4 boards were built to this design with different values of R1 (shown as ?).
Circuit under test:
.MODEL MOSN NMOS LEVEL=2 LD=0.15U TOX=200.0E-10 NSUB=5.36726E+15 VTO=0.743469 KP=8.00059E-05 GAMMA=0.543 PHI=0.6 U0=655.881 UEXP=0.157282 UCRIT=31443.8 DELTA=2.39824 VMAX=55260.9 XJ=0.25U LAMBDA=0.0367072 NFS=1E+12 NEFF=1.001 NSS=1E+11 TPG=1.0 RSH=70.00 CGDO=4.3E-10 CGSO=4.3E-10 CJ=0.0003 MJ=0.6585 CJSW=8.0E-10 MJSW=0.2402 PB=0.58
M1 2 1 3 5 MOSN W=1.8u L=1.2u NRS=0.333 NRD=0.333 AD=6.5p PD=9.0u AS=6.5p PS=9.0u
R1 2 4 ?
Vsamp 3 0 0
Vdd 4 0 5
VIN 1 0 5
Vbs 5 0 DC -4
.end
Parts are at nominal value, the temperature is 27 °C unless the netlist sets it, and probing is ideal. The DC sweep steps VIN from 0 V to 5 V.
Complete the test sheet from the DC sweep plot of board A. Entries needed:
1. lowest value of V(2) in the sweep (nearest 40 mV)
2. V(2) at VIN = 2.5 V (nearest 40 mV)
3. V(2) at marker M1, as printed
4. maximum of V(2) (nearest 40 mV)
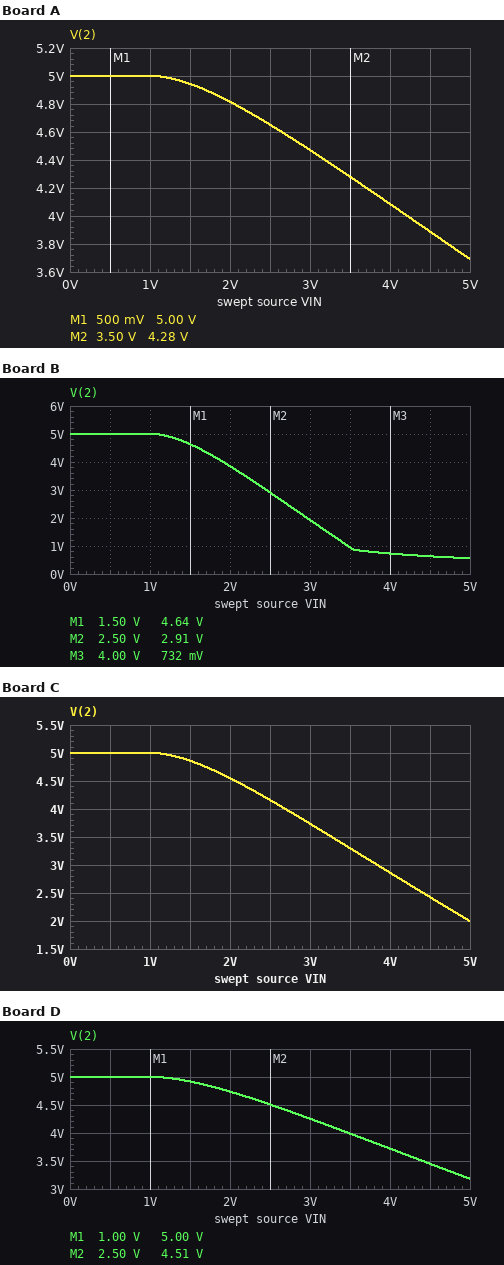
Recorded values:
3.68 V
4.64 V
5.00 V
5.00 V
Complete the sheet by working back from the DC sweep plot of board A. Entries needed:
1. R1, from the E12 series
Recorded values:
3.3 kΩ
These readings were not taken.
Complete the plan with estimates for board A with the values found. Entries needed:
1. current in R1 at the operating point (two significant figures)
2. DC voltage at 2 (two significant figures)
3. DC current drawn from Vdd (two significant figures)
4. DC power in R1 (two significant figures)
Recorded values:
400 µA
3.7 V
400 µA
520 µW
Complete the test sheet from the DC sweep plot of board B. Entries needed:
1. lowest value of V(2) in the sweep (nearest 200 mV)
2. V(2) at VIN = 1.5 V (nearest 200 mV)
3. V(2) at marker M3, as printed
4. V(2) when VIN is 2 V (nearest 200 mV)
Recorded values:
600 mV
4.6 V
732 mV
3.8 V
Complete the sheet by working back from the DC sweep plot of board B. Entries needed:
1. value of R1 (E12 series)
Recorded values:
22 kΩ
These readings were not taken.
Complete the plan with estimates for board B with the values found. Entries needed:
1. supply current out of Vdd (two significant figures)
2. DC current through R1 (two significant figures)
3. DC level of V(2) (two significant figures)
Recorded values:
200 µA
200 µA
560 mV
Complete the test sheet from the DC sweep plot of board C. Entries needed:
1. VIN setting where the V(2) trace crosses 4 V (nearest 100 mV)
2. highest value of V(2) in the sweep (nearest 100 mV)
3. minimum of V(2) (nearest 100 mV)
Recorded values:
2.7 V
5.0 V
2.0 V
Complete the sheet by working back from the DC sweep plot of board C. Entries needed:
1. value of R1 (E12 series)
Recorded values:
8.2 kΩ
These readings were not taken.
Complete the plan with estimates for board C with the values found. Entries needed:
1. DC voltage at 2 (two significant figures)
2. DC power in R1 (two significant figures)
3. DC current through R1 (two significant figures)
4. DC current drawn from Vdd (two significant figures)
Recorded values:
2.0 V
1.1 mW
370 µA
370 µA
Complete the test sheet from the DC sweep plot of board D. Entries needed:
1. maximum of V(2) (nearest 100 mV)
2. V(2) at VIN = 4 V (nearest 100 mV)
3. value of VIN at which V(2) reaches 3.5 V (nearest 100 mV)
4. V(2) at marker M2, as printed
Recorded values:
5.0 V
3.7 V
4.4 V
4.51 V
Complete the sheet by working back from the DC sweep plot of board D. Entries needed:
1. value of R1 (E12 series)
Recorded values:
4.7 kΩ
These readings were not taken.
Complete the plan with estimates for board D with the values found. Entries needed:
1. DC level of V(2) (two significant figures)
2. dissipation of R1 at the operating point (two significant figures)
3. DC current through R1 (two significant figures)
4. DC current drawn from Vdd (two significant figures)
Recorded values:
3.2 V
700 µW
390 µA
390 µA
